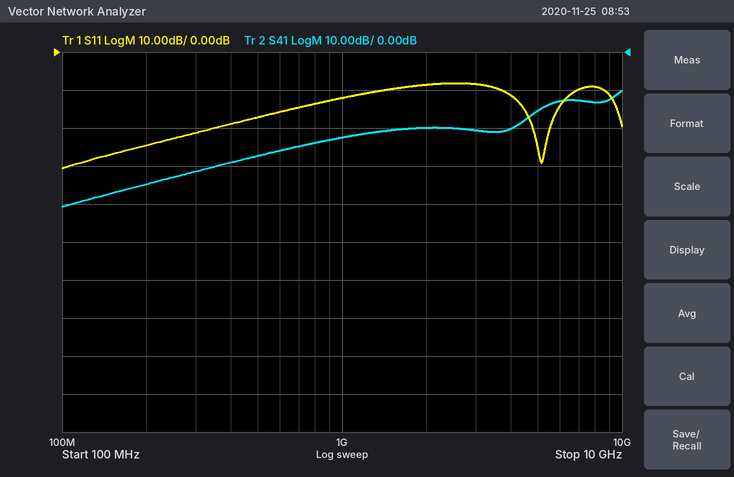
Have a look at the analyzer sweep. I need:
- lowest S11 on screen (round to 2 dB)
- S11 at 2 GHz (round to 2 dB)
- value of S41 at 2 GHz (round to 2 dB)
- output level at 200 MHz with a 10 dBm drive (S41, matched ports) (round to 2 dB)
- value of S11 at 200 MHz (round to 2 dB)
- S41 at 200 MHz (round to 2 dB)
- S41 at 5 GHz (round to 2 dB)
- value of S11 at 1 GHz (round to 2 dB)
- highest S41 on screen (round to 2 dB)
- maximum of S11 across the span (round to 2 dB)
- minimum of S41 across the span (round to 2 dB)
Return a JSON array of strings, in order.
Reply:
["-30 dB", "-8 dB", "-20 dB", "-24 dBm", "-24 dB", "-34 dB", "-16 dB", "-12 dB", "-10 dB", "-8 dB", "-40 dB"]
